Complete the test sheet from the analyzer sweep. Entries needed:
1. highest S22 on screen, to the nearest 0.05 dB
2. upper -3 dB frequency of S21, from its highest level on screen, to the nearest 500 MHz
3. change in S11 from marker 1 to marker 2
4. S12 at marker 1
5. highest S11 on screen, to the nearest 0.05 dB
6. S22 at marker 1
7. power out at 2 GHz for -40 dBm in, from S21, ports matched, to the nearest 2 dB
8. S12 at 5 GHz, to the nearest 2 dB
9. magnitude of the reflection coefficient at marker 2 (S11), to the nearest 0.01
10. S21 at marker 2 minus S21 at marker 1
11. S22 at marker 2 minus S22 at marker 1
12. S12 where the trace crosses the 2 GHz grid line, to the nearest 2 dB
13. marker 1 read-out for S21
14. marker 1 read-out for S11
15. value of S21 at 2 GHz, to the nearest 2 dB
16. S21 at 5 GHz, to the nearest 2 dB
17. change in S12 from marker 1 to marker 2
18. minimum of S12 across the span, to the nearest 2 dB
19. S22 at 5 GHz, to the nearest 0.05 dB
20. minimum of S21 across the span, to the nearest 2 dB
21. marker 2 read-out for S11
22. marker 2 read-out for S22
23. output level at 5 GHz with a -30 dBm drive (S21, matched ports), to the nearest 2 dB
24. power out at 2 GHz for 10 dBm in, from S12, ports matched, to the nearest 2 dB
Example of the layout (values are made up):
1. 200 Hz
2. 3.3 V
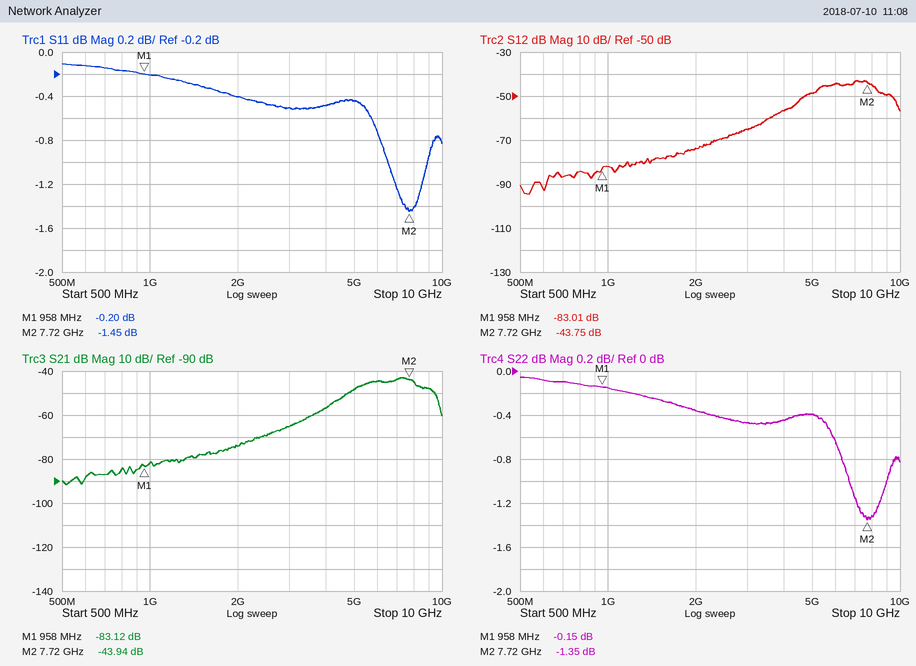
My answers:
1. -0.05 dB
2. 8.0 GHz
3. -1.25 dB
4. -83.01 dB
5. -0.10 dB
6. -0.15 dB
7. -114 dBm
8. -48 dB
9. 0.85
10. 39.18 dB
11. -1.20 dB
12. -74 dB
13. -83.12 dB
14. -0.20 dB
15. -74 dB
16. -48 dB
17. 39.26 dB
18. -94 dB
19. -0.40 dB
20. -92 dB
21. -1.45 dB
22. -1.35 dB
23. -78 dBm
24. -64 dBm
